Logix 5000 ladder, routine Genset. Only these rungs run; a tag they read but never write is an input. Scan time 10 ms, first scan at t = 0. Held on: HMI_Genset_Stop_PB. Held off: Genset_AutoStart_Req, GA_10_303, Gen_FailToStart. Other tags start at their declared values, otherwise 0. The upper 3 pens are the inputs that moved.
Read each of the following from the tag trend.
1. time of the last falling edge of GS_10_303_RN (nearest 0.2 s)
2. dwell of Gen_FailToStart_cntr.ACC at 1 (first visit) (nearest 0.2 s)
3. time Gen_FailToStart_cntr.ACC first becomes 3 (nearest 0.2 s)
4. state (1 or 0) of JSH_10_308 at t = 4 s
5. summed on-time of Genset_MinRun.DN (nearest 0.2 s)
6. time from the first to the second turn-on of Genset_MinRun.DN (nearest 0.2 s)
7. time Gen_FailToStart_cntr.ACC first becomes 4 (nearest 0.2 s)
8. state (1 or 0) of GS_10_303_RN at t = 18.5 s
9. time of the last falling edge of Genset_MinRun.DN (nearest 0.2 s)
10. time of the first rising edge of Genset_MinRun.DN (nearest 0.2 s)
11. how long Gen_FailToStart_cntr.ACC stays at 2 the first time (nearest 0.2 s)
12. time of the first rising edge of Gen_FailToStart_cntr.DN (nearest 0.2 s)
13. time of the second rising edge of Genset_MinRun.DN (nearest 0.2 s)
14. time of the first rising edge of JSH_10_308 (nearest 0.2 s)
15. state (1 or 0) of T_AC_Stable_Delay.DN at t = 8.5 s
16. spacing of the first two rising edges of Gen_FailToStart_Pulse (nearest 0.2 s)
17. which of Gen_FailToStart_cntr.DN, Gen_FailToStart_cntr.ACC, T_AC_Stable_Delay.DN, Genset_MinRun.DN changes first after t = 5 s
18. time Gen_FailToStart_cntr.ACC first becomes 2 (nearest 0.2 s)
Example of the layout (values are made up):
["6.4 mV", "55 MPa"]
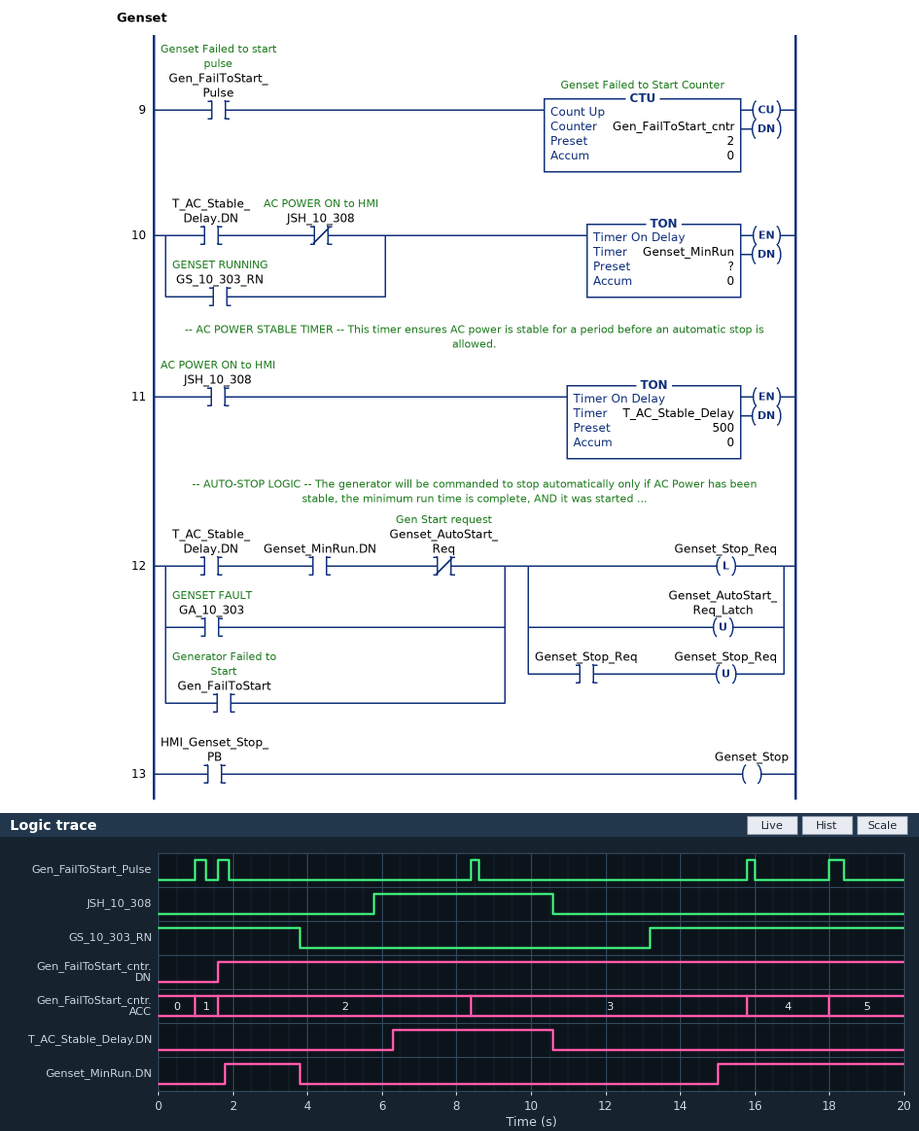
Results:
["3.8 s", "0.6 s", "8.4 s", "0", "7.0 s", "13.2 s", "15.8 s", "1", "3.8 s", "1.8 s", "6.8 s", "1.6 s", "15.0 s", "5.8 s", "1", "0.6 s", "T_AC_Stable_Delay.DN", "1.6 s"]
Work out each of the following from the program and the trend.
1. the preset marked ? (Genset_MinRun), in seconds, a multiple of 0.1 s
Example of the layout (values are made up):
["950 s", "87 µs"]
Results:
["1.8 s"]
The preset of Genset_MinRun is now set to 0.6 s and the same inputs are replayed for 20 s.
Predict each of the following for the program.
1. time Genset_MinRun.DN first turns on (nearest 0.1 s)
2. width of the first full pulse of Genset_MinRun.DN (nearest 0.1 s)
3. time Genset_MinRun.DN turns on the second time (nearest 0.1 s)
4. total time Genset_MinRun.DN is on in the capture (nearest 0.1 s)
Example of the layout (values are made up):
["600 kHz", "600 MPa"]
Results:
["0.6 s", "3.2 s", "13.8 s", "9.4 s"]
